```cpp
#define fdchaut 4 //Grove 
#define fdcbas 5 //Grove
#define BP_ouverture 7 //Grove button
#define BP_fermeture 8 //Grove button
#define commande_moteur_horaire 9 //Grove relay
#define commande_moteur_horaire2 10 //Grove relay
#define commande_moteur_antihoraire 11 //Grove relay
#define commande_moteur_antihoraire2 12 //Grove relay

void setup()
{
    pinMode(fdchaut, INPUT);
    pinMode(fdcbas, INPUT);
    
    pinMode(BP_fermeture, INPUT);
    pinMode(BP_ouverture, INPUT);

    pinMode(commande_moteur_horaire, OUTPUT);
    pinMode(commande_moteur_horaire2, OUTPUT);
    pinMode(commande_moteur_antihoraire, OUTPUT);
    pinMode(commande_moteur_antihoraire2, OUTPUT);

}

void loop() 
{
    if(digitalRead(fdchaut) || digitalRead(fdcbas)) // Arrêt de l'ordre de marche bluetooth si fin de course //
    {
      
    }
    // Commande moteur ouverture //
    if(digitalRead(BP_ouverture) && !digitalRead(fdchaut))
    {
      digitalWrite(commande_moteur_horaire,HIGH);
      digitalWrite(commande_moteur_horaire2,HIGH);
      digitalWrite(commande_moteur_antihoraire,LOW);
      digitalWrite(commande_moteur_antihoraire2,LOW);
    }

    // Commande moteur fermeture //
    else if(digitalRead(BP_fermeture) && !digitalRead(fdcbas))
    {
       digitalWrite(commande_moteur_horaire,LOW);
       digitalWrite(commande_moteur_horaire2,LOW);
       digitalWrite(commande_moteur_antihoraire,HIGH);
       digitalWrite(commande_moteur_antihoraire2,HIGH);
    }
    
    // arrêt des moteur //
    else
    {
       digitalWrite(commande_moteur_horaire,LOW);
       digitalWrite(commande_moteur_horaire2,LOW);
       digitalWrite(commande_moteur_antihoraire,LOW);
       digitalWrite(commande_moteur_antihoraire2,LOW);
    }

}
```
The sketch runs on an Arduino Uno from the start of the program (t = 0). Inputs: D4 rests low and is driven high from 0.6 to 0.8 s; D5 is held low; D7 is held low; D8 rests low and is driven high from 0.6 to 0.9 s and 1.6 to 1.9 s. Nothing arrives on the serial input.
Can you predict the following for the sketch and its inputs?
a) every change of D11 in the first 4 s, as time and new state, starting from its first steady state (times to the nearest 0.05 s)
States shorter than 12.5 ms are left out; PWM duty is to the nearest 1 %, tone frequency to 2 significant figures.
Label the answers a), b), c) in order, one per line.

a) 0 s low; 0.6 s high; 0.9 s low; 1.6 s high; 1.9 s low
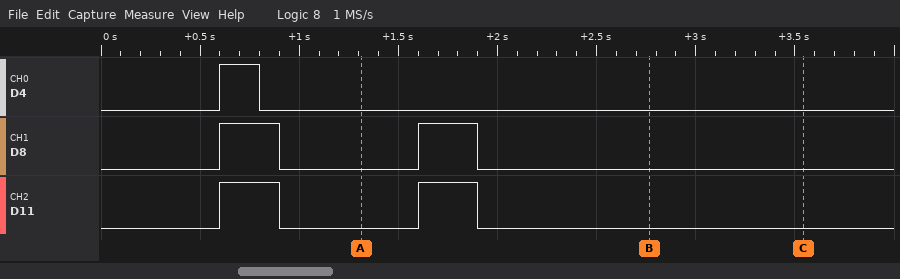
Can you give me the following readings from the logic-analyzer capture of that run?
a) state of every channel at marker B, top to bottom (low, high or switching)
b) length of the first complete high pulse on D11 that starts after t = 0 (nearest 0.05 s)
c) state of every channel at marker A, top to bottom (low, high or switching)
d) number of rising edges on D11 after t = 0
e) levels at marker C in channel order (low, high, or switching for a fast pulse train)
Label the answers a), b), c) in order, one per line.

a) D4 low, D8 low, D11 low
b) 0.30 s
c) D4 low, D8 low, D11 low
d) 2
e) D4 low, D8 low, D11 low
